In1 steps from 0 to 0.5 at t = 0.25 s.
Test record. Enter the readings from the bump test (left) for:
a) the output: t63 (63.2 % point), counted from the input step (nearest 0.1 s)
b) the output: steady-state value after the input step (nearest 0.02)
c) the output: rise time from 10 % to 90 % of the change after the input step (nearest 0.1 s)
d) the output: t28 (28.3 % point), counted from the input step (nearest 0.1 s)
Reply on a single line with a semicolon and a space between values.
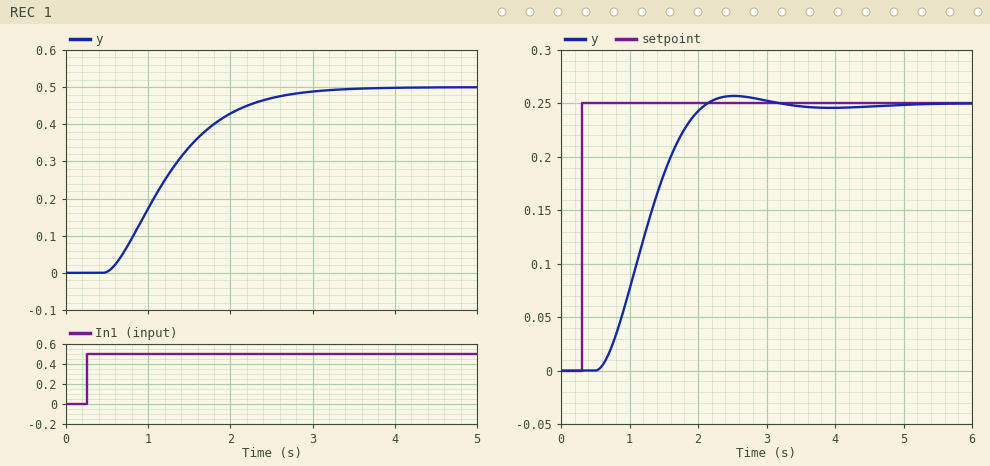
1.2 s; 0.50; 1.5 s; 0.7 s
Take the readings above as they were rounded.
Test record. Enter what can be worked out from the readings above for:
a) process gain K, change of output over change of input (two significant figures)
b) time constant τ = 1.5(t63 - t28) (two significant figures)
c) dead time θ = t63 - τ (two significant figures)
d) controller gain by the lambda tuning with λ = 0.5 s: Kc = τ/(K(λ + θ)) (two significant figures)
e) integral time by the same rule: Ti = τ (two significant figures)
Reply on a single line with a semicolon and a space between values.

1.0; 0.75 s; 0.45 s; 0.79; 0.75 s
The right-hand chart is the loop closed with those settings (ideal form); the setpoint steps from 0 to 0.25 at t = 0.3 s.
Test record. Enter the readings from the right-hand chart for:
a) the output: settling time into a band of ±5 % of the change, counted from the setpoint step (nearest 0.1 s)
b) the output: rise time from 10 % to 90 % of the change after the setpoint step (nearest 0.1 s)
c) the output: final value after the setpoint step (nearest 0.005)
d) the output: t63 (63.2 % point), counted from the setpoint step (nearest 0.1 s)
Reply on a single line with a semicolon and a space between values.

1.6 s; 1.0 s; 0.250; 1.1 s
